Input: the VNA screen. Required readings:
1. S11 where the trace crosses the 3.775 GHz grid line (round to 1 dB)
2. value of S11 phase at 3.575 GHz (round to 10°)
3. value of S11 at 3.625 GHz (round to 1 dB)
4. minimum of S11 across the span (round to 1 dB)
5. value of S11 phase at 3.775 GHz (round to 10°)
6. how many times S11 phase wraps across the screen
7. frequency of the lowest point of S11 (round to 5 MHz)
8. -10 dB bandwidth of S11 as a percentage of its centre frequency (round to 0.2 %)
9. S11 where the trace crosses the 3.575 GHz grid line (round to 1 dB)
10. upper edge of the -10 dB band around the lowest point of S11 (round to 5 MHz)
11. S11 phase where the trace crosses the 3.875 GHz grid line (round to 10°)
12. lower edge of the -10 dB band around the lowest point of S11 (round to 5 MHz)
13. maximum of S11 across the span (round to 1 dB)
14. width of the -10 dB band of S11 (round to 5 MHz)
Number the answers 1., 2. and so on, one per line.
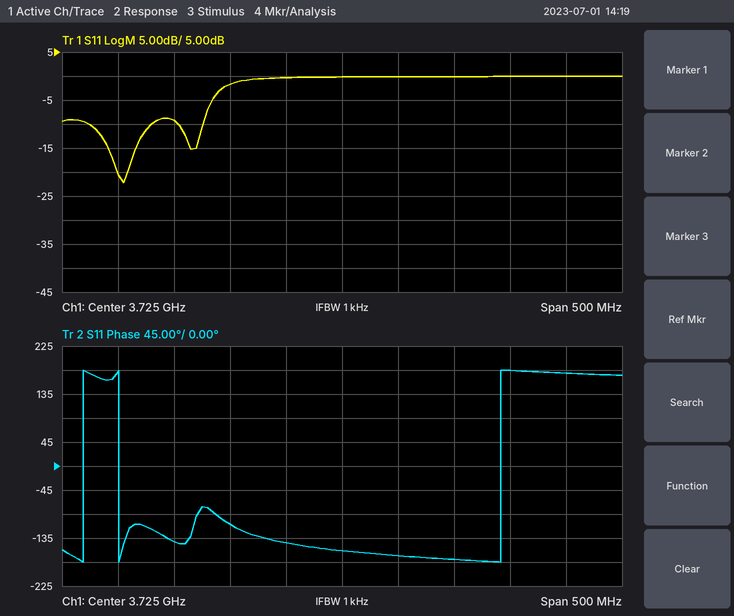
1. 0 dB
2. -140°
3. -2 dB
4. -22 dB
5. -170°
6. 3
7. 3.530 GHz
8. 1.6 %
9. -9 dB
10. 3.555 GHz
11. 180°
12. 3.500 GHz
13. 0 dB
14. 55 MHz
